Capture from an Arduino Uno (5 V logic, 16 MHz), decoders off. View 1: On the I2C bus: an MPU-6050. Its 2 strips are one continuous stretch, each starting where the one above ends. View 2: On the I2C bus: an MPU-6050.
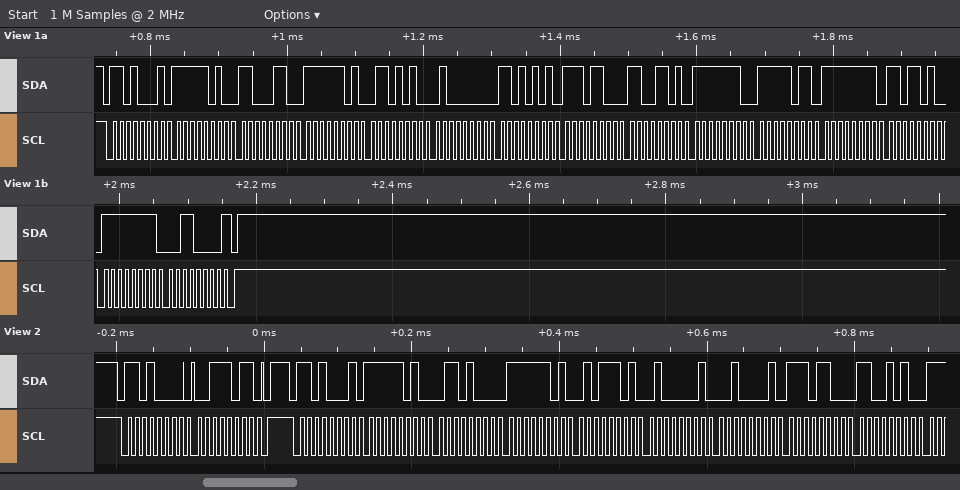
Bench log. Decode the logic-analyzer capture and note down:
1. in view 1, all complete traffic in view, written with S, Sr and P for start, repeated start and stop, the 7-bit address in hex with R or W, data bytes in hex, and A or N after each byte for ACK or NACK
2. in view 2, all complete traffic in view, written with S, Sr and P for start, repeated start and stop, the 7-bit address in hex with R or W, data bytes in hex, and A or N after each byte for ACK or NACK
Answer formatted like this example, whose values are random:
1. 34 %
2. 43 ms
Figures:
1. S 68R A FA A C6 A FD A 6A A 40 A D5 A EC A CD A FE A FB A FF A DA A FF A 30 N P
2. S 68W A 3B A P S 68R A FA A 68 A FD A 5D A 41 A 21 A EC A CA A
